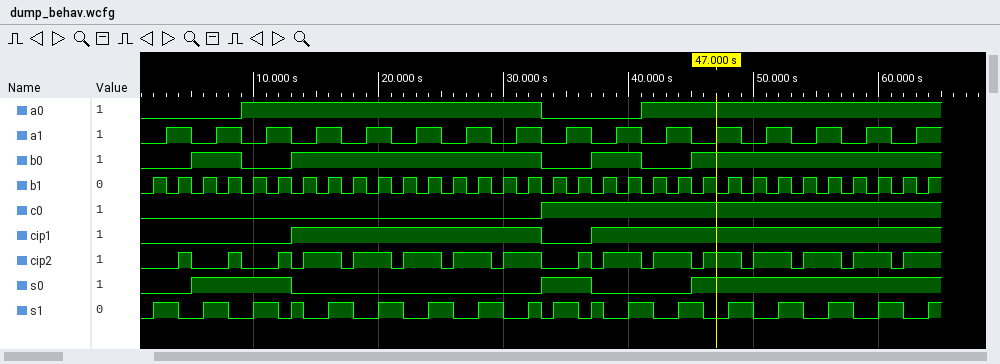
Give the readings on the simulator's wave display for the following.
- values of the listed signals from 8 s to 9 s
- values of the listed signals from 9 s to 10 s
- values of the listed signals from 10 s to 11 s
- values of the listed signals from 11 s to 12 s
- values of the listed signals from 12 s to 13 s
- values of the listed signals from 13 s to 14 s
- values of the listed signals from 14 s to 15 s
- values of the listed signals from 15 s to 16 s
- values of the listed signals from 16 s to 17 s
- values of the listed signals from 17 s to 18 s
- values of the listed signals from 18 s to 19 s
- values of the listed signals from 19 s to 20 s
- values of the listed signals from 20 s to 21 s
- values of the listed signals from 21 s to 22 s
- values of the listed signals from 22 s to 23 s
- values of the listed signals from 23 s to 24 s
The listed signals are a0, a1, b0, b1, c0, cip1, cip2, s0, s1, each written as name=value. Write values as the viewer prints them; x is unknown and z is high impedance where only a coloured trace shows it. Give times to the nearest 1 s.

a0=0, a1=1, b0=1, b1=1, c0=0, cip1=0, cip2=1, s0=1, s1=0
a0=1, a1=0, b0=0, b1=0, c0=0, cip1=0, cip2=0, s0=1, s1=0
a0=1, a1=0, b0=0, b1=1, c0=0, cip1=0, cip2=0, s0=1, s1=1
a0=1, a1=1, b0=0, b1=0, c0=0, cip1=0, cip2=0, s0=1, s1=1
a0=1, a1=1, b0=0, b1=1, c0=0, cip1=0, cip2=1, s0=1, s1=0
a0=1, a1=0, b0=1, b1=0, c0=0, cip1=1, cip2=0, s0=0, s1=1
a0=1, a1=0, b0=1, b1=1, c0=0, cip1=1, cip2=1, s0=0, s1=0
a0=1, a1=1, b0=1, b1=0, c0=0, cip1=1, cip2=1, s0=0, s1=0
a0=1, a1=1, b0=1, b1=1, c0=0, cip1=1, cip2=1, s0=0, s1=1
a0=1, a1=0, b0=1, b1=0, c0=0, cip1=1, cip2=0, s0=0, s1=1
a0=1, a1=0, b0=1, b1=1, c0=0, cip1=1, cip2=1, s0=0, s1=0
a0=1, a1=1, b0=1, b1=0, c0=0, cip1=1, cip2=1, s0=0, s1=0
a0=1, a1=1, b0=1, b1=1, c0=0, cip1=1, cip2=1, s0=0, s1=1
a0=1, a1=0, b0=1, b1=0, c0=0, cip1=1, cip2=0, s0=0, s1=1
a0=1, a1=0, b0=1, b1=1, c0=0, cip1=1, cip2=1, s0=0, s1=0
a0=1, a1=1, b0=1, b1=0, c0=0, cip1=1, cip2=1, s0=0, s1=0
